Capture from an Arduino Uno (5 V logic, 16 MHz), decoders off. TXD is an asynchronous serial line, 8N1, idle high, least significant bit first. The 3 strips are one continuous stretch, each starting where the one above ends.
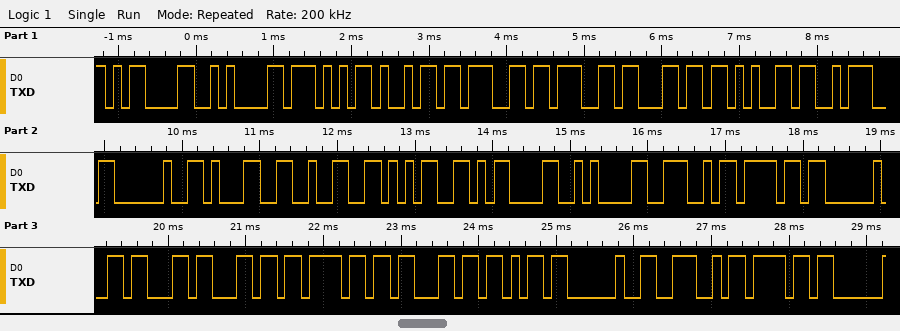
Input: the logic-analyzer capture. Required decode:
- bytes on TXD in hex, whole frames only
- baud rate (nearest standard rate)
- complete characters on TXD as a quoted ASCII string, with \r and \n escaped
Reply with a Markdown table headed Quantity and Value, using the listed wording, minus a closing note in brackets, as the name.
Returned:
| Quantity | Value |
|---|---|
| bytes on TXD in hex, whole frames only | 0x0D 0x0A 0x57 0x69 0x67 0x67 0x6C 0x65 0x3A 0x20 0x31 0x32 0x35 0x0D 0x0A 0x4E 0x6F 0x20 0x63 0x6C 0x6F 0x63 0x6B 0x20 0x4E 0x6F |
| baud rate | 9600 baud |
| complete characters on TXD as a quoted ASCII string, with \r and \n escaped | "\r\nWiggle: 125\r\nNo clock No" |
